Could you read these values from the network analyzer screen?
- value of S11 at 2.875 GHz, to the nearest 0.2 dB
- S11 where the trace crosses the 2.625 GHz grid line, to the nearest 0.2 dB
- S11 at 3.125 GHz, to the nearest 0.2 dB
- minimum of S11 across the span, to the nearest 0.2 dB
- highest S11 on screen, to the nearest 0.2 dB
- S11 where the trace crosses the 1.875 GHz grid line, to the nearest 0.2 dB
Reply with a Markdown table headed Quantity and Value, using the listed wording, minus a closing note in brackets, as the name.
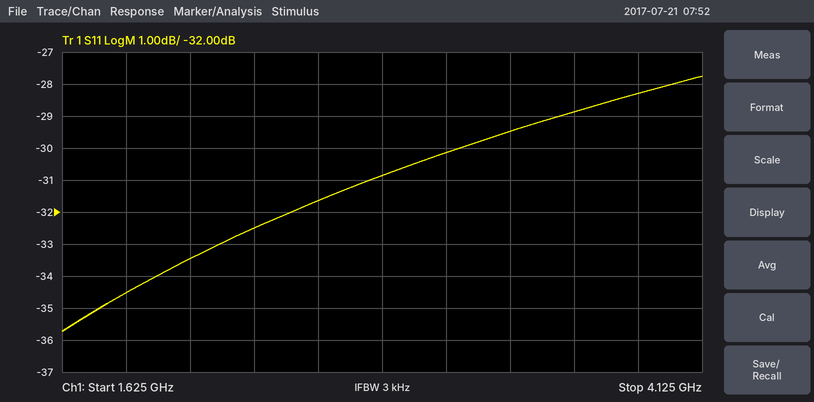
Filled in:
| Quantity | Value |
|---|---|
| value of S11 at 2.875 GHz, to the nearest 0.2 dB | -30.8 dB |
| S11 where the trace crosses the 2.625 GHz grid line, to the nearest 0.2 dB | -31.6 dB |
| S11 at 3.125 GHz, to the nearest 0.2 dB | -30.2 dB |
| minimum of S11 across the span, to the nearest 0.2 dB | -35.8 dB |
| highest S11 on screen, to the nearest 0.2 dB | -27.8 dB |
| S11 where the trace crosses the 1.875 GHz grid line, to the nearest 0.2 dB | -34.6 dB |
